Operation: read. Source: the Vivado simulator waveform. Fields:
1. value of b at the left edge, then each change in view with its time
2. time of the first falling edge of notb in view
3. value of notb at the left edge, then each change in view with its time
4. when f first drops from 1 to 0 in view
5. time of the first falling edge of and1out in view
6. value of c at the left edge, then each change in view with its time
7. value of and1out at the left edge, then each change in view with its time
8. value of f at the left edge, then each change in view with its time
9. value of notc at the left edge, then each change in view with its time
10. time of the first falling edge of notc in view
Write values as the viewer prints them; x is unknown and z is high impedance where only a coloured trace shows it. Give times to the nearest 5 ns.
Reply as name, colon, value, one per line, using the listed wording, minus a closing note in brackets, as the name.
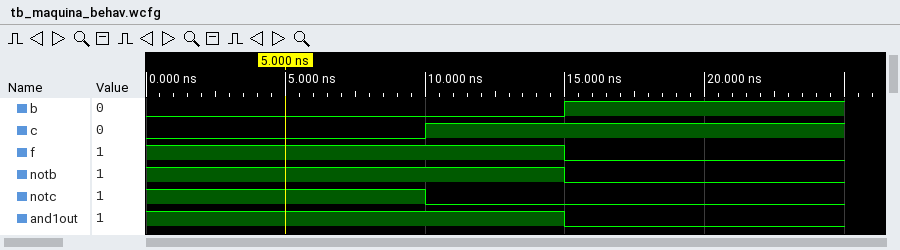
value of b at the left edge, then each change in view with its time: 0, 1 at 15 ns
time of the first falling edge of notb in view: 15 ns
value of notb at the left edge, then each change in view with its time: 1, 0 at 15 ns
when f first drops from 1 to 0 in view: 15 ns
time of the first falling edge of and1out in view: 15 ns
value of c at the left edge, then each change in view with its time: 0, 1 at 10 ns
value of and1out at the left edge, then each change in view with its time: 1, 0 at 15 ns
value of f at the left edge, then each change in view with its time: 1, 0 at 15 ns
value of notc at the left edge, then each change in view with its time: 1, 0 at 10 ns
time of the first falling edge of notc in view: 10 ns
